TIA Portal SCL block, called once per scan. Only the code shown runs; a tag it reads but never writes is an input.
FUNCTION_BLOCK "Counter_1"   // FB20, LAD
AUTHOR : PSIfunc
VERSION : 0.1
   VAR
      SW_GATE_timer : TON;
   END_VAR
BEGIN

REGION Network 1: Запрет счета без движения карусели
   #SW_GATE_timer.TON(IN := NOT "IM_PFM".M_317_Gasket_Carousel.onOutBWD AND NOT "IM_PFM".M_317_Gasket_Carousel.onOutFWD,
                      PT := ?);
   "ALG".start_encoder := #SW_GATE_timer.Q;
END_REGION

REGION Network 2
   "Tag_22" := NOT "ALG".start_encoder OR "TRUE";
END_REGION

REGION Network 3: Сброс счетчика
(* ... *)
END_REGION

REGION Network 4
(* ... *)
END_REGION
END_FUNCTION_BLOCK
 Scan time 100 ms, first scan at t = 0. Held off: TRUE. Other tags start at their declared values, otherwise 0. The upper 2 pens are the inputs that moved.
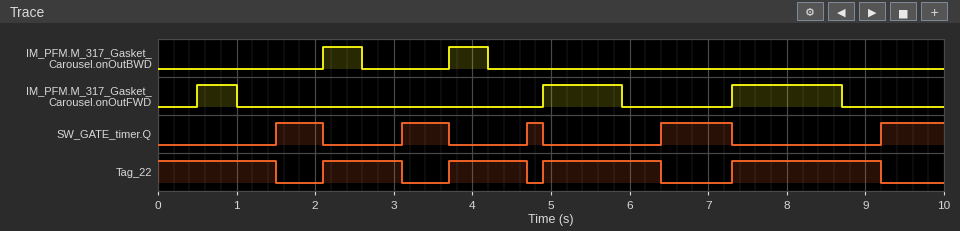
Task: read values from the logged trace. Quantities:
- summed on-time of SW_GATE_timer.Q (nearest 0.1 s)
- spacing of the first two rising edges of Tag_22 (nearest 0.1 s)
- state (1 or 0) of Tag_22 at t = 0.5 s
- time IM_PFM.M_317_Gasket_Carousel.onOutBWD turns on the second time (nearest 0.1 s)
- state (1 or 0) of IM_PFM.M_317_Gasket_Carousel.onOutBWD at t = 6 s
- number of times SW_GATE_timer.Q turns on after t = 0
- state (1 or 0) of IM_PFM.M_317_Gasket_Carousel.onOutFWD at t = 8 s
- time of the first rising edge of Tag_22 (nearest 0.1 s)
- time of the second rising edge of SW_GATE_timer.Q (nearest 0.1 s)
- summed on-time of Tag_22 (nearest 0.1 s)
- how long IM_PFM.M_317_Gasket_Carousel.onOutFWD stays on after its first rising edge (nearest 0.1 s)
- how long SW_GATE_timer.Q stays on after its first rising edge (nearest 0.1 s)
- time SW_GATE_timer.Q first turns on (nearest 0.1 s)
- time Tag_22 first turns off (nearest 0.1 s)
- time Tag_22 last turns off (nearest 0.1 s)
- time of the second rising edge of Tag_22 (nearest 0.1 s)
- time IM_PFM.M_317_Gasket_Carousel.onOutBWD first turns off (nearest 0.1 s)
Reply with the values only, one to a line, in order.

3.1 s
1.6 s
1
3.7 s
0
5
1
2.1 s
3.1 s
6.9 s
0.5 s
0.6 s
1.5 s
1.5 s
9.2 s
3.7 s
2.6 s
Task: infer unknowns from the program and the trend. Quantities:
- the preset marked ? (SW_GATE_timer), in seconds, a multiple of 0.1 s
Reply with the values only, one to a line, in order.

0.5 s
